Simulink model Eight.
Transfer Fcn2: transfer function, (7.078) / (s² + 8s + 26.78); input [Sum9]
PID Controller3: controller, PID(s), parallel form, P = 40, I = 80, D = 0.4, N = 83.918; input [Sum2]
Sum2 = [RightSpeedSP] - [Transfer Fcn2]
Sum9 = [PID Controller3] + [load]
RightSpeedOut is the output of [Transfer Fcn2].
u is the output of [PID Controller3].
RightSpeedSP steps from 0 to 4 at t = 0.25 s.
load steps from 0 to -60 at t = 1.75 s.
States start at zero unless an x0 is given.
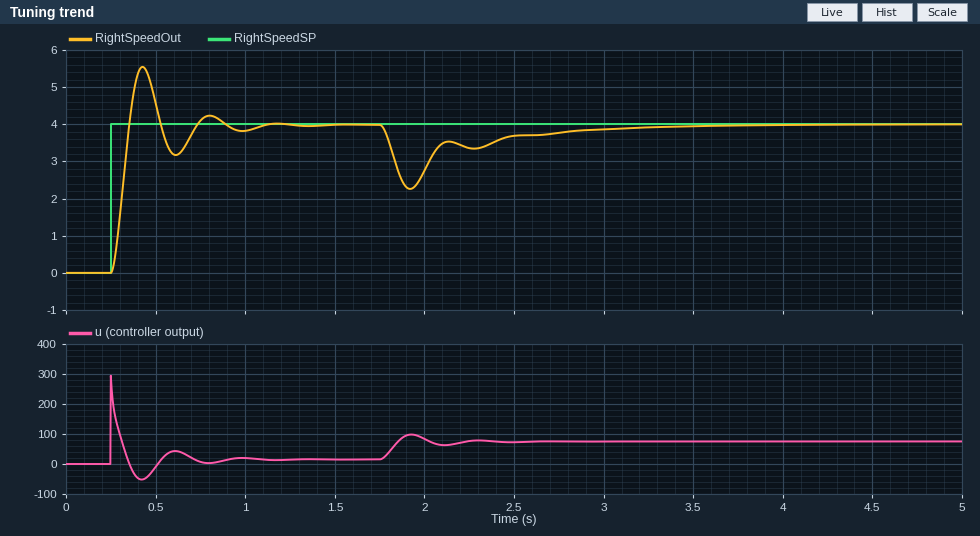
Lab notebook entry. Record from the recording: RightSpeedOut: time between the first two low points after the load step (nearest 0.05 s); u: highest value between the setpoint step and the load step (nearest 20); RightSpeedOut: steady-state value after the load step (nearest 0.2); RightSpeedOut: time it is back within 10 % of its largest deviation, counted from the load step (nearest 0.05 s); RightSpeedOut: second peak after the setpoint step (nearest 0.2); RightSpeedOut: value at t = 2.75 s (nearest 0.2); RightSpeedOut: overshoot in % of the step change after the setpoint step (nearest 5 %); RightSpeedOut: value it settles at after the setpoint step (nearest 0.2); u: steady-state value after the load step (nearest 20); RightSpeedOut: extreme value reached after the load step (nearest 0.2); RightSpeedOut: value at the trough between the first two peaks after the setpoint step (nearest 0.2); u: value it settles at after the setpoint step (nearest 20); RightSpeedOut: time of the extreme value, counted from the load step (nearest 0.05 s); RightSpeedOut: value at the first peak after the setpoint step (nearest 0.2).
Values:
0.35 s
300
4.0
1.10 s
4.2
3.8
40 %
4.0
80
2.2
3.2
20
0.15 s
5.6
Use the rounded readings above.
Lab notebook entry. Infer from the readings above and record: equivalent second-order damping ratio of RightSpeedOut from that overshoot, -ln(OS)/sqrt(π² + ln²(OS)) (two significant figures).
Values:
0.28
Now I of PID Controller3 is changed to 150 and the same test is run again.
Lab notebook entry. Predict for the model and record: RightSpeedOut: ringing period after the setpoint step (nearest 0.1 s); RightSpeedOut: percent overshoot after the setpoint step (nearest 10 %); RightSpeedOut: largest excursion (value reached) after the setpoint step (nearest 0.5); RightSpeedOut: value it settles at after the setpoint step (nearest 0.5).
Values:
0.4 s
50 %
6.0
4.0
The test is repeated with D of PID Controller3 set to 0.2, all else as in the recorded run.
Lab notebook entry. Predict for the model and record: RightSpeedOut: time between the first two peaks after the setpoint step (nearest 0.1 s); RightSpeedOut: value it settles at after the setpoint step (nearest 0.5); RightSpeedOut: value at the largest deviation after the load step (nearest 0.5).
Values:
0.4 s
4.0
2.0
